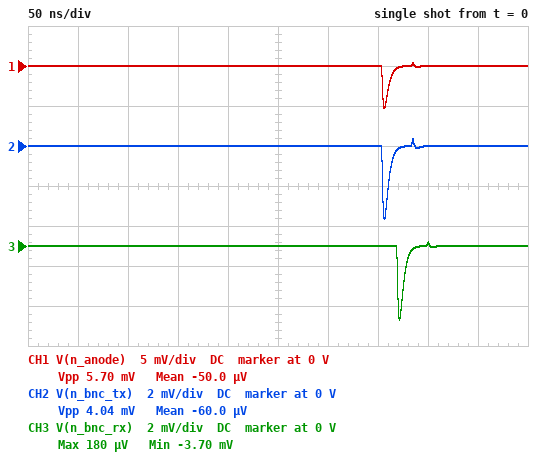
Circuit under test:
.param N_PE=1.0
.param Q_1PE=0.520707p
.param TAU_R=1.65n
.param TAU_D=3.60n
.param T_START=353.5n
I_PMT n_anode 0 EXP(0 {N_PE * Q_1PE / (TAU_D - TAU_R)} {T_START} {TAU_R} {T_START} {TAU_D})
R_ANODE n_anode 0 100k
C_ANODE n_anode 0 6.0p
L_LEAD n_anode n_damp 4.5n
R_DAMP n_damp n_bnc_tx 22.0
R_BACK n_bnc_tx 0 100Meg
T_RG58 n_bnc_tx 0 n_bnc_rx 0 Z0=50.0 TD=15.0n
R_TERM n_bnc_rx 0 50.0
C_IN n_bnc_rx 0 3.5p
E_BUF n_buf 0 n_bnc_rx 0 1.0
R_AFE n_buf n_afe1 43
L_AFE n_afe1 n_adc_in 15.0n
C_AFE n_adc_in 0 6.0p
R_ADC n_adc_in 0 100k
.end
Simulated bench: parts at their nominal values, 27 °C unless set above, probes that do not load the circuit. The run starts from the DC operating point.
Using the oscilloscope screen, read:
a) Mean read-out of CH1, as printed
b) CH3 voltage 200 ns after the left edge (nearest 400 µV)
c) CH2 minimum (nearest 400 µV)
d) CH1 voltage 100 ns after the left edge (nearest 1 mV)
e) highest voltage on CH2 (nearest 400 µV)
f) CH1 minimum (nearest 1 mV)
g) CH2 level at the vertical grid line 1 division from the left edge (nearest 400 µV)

-50.0 µV
0 V
-3.6 mV
0 V
400 µV
-5 mV
0 V
